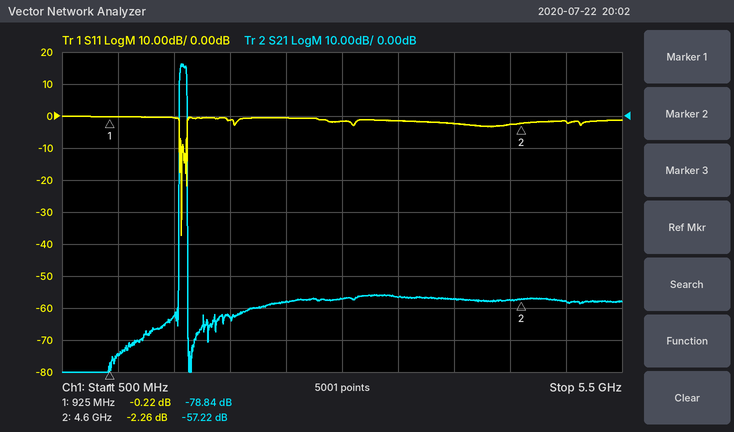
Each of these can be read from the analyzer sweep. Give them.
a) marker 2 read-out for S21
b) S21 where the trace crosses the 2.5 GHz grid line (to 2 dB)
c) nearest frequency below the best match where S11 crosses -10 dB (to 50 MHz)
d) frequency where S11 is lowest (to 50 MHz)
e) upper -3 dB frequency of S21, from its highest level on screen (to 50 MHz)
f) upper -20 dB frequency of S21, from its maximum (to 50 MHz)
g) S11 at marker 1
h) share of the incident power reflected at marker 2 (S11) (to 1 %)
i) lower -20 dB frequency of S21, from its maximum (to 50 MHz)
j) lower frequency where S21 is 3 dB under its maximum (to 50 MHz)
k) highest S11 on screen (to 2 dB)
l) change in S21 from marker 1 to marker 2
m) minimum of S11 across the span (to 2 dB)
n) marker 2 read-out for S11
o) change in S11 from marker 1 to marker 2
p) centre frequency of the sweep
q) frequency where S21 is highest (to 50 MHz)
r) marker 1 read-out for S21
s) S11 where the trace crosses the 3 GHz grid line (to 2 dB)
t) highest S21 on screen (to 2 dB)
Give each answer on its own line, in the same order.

-57.22 dB
-58 dB
1.55 GHz
1.55 GHz
1.60 GHz
1.60 GHz
-0.22 dB
59 %
1.55 GHz
1.55 GHz
0 dB
21.62 dB
-38 dB
-2.26 dB
-2.04 dB
3 GHz
1.55 GHz
-78.84 dB
-2 dB
16 dB
